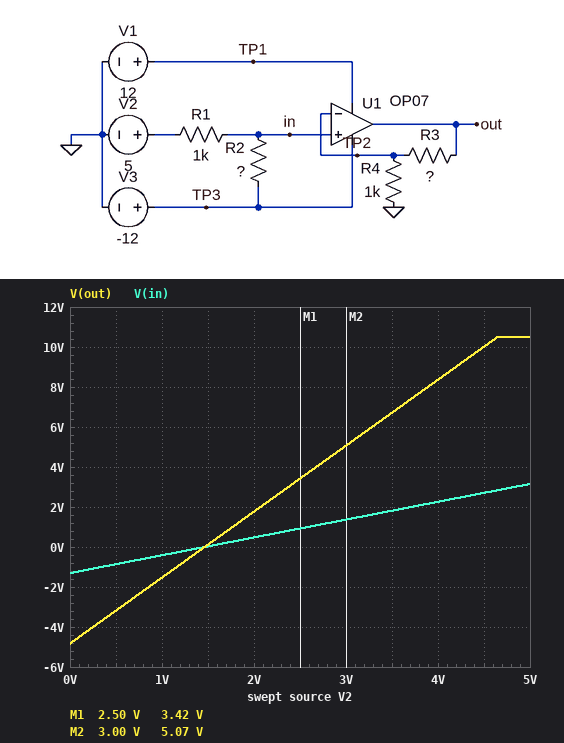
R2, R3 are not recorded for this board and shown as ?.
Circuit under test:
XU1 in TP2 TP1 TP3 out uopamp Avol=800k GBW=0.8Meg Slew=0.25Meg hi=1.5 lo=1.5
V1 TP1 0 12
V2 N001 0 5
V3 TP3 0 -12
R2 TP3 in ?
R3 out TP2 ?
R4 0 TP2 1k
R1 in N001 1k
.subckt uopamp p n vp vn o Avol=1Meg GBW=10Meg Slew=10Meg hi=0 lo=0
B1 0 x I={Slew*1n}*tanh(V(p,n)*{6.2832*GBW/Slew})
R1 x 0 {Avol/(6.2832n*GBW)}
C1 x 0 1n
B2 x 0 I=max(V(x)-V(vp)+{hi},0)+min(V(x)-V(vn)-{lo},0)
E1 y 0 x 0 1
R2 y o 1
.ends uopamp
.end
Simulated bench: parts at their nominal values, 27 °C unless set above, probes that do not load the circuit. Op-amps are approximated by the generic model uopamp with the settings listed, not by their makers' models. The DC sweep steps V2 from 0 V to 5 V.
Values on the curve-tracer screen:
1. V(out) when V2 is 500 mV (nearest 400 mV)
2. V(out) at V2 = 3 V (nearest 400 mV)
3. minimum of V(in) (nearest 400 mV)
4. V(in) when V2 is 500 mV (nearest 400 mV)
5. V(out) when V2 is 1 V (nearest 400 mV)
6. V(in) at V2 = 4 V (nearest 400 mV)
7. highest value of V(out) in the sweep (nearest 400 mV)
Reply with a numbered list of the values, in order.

1. -3.2 V
2. 5.2 V
3. -1.2 V
4. -800 mV
5. -1.6 V
6. 2.4 V
7. 10.4 V
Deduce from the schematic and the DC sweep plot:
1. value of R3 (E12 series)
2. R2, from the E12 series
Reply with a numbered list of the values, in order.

1. 2.7 kΩ
2. 8.2 kΩ
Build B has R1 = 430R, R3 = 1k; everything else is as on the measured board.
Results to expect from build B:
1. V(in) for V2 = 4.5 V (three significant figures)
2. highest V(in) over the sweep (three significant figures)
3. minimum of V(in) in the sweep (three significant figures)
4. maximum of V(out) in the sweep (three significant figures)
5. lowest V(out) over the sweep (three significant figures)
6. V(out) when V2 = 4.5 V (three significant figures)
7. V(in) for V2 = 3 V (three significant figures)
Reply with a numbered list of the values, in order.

1. 3.68 V
2. 4.15 V
3. -598 mV
4. 8.31 V
5. -1.20 V
6. 7.36 V
7. 2.25 V
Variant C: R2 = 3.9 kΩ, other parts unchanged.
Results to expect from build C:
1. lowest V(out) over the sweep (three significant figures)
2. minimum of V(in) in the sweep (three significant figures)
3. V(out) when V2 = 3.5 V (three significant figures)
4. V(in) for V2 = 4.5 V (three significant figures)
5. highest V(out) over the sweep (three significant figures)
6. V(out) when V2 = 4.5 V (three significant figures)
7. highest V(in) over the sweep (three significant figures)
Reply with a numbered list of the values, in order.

1. -9.06 V
2. -2.45 V
3. 1.25 V
4. 1.13 V
5. 5.66 V
6. 4.19 V
7. 1.53 V
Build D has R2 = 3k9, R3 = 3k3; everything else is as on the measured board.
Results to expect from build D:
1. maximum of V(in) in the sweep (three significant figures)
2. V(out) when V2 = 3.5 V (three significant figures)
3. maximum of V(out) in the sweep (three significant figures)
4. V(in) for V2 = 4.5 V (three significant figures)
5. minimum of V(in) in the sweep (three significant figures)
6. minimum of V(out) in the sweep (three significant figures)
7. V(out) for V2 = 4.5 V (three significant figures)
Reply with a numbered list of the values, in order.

1. 1.53 V
2. 1.45 V
3. 6.58 V
4. 1.13 V
5. -2.45 V
6. -10.5 V
7. 4.87 V
